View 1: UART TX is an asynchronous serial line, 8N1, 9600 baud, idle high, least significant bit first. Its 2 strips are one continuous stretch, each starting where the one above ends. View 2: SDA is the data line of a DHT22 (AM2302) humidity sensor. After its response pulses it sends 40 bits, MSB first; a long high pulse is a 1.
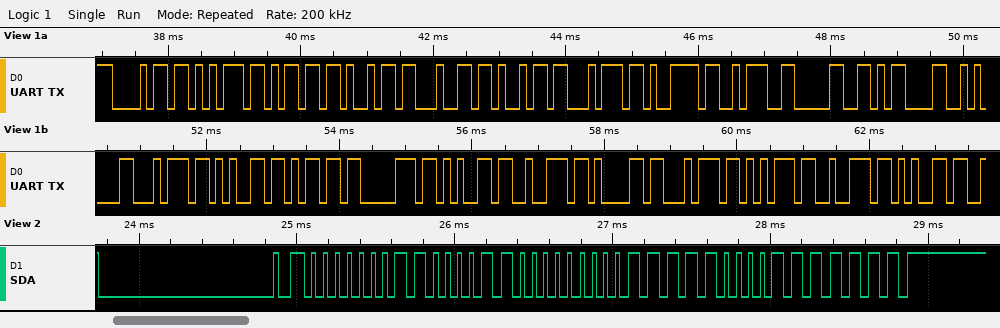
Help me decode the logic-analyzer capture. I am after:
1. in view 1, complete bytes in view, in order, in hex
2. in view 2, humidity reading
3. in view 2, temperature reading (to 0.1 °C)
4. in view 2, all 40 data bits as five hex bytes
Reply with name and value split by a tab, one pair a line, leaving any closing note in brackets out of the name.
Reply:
in view 1, complete bytes in view, in order, in hex	0x68 0x75 0x6D 0x69 0x64 0x69 0x74 0x79 0x3A 0x30 0x0D 0x0A 0x74 0x65 0x6D 0x70 0x65 0x72 0x61 0x74 0x75 0x72 0x65
in view 2, humidity reading	39.0 %
in view 2, temperature reading	24.8 °C
in view 2, all 40 data bits as five hex bytes	01 86 00 F8 7F
